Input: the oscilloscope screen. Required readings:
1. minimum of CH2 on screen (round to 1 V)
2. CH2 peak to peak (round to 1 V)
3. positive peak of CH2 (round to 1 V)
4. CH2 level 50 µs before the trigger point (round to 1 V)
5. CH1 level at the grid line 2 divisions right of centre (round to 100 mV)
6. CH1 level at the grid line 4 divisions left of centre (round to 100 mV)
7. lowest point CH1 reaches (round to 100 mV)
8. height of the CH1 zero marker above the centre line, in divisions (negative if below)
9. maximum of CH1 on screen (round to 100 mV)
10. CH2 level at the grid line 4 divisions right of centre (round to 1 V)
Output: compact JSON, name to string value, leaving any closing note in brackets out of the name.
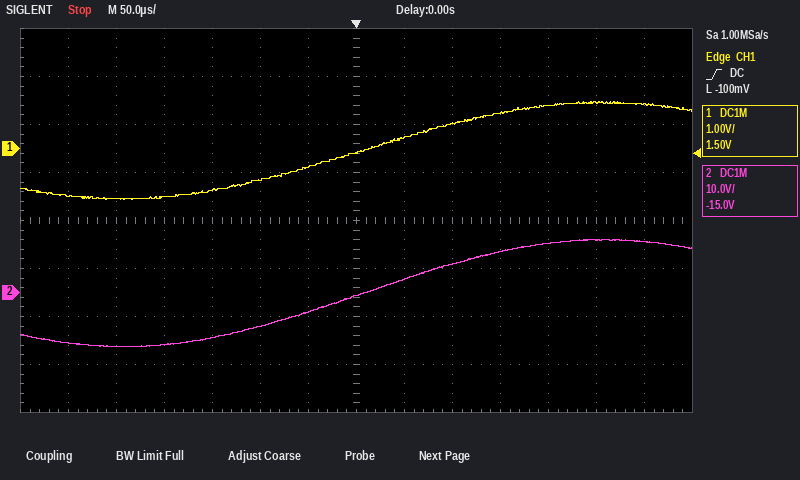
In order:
{"minimum of CH2 on screen": "-11 V", "CH2 peak to peak": "22 V", "positive peak of CH2": "11 V", "CH2 level 50 µs before the trigger point": "-4 V", "CH1 level at the grid line 2 divisions right of centre": "500 mV", "CH1 level at the grid line 4 divisions left of centre": "-1.0 V", "lowest point CH1 reaches": "-1.1 V", "height of the CH1 zero marker above the centre line, in divisions": "+1.5 div", "maximum of CH1 on screen": "1.0 V", "CH2 level at the grid line 4 divisions right of centre": "10 V"}
